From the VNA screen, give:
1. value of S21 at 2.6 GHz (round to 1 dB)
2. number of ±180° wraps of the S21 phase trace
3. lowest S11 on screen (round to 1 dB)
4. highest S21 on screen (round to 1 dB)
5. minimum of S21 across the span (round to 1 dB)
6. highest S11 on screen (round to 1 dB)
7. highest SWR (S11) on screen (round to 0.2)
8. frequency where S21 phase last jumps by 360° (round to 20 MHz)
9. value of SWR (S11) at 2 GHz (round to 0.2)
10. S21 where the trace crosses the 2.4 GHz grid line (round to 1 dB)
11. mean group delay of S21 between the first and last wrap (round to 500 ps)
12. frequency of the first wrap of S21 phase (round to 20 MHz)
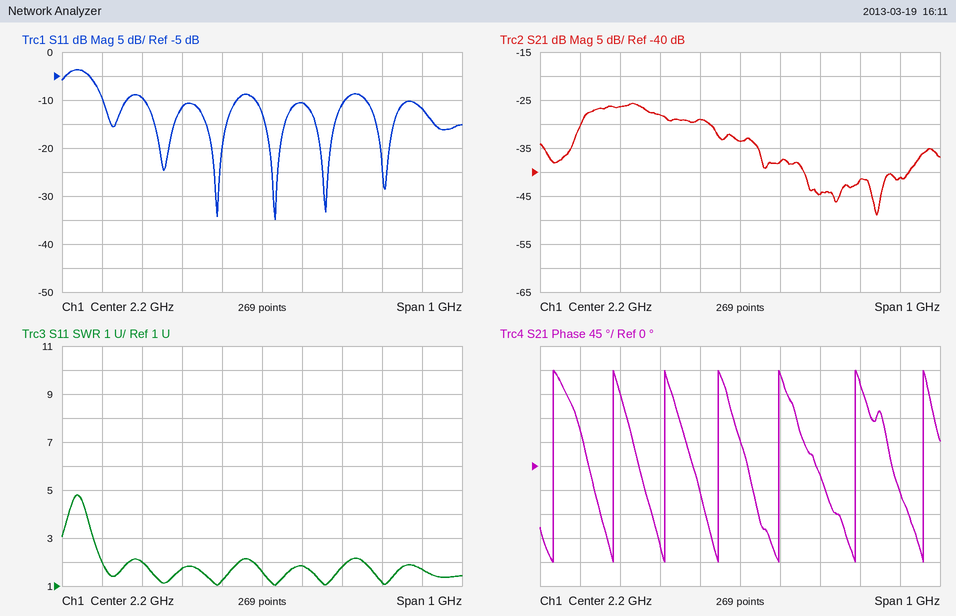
-41 dB
7
-35 dB
-26 dB
-49 dB
-4 dB
4.8
2.66 GHz
1.8
-45 dB
6.5 ns
1.74 GHz
